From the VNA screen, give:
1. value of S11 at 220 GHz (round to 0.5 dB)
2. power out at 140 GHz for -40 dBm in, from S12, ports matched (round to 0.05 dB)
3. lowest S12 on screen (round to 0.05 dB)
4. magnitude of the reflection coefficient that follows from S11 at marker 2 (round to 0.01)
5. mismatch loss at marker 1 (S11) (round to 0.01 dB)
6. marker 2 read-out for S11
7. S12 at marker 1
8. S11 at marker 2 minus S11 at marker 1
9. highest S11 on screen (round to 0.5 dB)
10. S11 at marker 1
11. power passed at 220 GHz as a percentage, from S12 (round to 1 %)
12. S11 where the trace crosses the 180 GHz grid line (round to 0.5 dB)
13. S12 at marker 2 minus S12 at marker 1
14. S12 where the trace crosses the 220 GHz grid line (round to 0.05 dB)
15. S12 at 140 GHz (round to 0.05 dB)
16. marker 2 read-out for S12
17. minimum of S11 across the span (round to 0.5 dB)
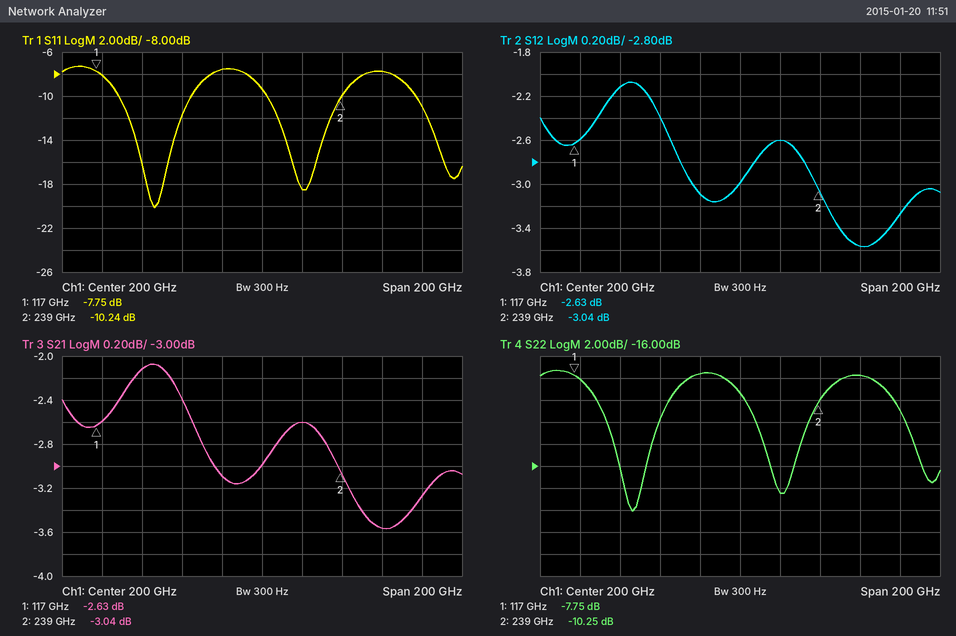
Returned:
-18.5 dB
-42.10 dBm
-3.55 dB
0.31
0.80 dB
-10.24 dB
-2.63 dB
-2.49 dB
-7.5 dB
-7.75 dB
55 %
-7.5 dB
-0.41 dB
-2.60 dB
-2.10 dB
-3.04 dB
-20.0 dB
